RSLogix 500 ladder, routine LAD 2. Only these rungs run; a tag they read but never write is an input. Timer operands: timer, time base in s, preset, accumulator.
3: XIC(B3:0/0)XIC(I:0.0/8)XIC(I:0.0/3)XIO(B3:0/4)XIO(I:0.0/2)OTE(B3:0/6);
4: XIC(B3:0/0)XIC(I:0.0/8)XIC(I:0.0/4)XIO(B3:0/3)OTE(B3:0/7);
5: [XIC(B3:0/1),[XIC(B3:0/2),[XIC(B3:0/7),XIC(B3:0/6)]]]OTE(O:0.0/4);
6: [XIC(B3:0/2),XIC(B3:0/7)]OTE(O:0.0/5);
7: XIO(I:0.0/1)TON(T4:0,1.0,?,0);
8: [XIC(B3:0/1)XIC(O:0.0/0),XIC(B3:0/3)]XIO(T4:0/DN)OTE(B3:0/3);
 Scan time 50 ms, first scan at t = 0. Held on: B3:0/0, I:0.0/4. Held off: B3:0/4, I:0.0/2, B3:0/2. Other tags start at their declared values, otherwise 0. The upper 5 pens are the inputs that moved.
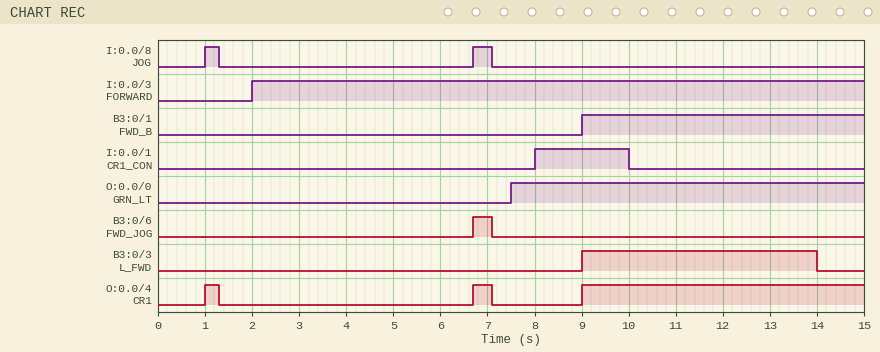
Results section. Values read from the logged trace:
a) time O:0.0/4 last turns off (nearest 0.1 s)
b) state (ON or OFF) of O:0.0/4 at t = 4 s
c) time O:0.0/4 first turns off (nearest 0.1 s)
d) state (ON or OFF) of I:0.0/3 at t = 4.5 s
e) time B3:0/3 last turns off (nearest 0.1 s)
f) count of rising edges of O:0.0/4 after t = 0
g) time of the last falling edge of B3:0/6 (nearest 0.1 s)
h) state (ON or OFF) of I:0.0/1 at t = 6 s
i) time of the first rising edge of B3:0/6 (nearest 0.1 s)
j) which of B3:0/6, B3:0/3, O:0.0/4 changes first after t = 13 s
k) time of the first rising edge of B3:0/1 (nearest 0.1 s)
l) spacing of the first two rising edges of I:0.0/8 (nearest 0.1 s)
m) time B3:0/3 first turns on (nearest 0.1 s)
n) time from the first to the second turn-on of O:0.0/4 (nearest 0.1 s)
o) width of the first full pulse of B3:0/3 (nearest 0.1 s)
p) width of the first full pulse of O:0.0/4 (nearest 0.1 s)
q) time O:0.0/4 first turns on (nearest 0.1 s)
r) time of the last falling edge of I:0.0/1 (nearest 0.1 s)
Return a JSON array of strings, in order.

["7.1 s", "OFF", "1.3 s", "ON", "14.0 s", "3", "7.1 s", "OFF", "6.7 s", "B3:0/3", "9.0 s", "5.7 s", "9.0 s", "5.7 s", "5.0 s", "0.3 s", "1.0 s", "10.0 s"]
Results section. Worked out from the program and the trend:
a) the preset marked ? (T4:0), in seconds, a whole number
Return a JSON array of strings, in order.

["4 s"]
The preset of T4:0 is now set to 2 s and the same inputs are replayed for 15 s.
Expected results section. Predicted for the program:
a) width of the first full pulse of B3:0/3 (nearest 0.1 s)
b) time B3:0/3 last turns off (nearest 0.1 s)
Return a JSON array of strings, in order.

["3.0 s", "12.0 s"]
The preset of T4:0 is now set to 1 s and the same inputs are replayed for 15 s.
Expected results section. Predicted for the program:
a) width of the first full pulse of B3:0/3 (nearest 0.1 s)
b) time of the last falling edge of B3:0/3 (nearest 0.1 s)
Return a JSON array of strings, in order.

["2.0 s", "11.0 s"]
